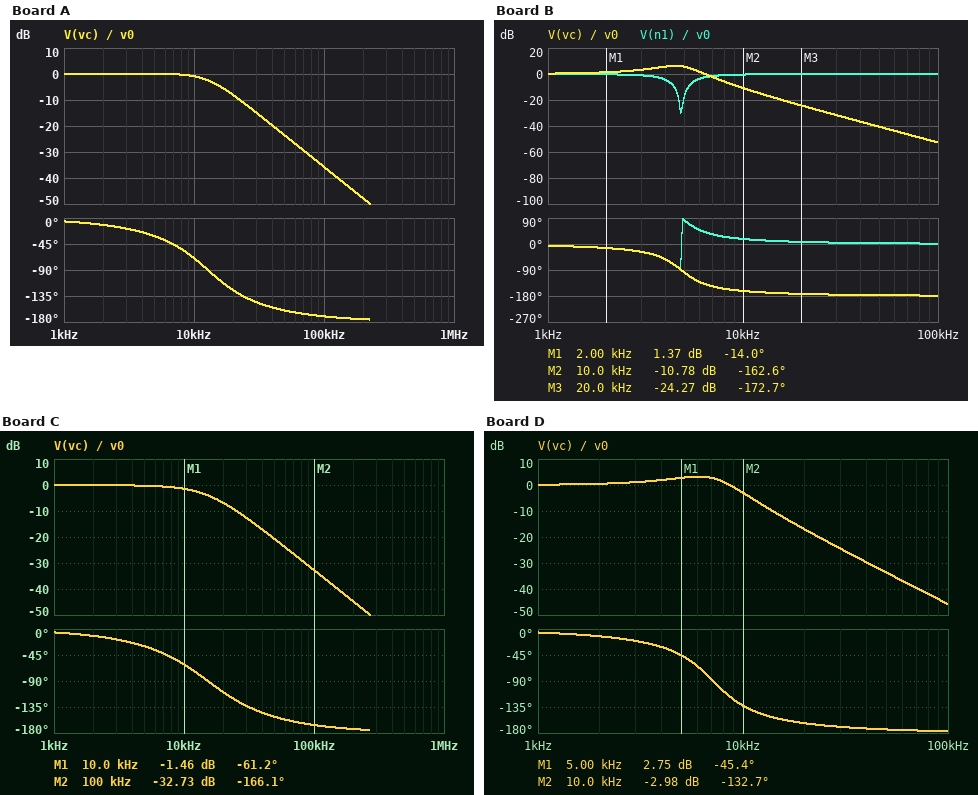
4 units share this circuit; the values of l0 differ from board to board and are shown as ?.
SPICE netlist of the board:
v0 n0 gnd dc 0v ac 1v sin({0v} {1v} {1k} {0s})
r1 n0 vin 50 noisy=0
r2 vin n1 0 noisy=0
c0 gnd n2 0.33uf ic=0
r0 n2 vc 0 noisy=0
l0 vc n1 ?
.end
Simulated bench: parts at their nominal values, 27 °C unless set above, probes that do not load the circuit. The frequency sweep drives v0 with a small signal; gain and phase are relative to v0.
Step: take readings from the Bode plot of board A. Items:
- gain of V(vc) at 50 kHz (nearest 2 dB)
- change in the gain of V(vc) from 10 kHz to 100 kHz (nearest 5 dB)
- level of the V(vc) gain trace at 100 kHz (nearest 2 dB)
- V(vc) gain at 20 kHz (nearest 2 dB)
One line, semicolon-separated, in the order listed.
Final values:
-24 dB; -35 dB; -36 dB; -8 dB
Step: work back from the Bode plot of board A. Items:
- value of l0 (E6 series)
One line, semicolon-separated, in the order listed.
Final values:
470 µH
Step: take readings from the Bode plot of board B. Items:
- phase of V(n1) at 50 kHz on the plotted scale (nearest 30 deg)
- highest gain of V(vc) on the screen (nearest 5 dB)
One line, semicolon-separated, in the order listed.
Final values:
0 deg; 5 dB
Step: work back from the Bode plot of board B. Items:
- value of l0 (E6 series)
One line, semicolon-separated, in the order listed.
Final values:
3.3 mH
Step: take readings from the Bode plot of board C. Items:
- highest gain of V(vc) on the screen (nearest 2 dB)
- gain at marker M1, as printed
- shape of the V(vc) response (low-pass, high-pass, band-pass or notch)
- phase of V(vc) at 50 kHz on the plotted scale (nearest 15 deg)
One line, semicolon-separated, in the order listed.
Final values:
0 dB; -1.46 dB; low-pass; -150 deg
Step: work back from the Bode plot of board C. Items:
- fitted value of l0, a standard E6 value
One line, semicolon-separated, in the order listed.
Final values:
330 µH
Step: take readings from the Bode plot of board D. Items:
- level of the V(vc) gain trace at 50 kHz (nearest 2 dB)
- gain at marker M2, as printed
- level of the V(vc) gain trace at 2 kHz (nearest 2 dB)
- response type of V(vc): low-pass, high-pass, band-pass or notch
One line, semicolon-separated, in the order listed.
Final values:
-34 dB; -2.98 dB; 0 dB; low-pass
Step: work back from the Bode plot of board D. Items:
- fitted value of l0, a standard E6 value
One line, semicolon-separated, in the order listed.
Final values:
1.5 mH
